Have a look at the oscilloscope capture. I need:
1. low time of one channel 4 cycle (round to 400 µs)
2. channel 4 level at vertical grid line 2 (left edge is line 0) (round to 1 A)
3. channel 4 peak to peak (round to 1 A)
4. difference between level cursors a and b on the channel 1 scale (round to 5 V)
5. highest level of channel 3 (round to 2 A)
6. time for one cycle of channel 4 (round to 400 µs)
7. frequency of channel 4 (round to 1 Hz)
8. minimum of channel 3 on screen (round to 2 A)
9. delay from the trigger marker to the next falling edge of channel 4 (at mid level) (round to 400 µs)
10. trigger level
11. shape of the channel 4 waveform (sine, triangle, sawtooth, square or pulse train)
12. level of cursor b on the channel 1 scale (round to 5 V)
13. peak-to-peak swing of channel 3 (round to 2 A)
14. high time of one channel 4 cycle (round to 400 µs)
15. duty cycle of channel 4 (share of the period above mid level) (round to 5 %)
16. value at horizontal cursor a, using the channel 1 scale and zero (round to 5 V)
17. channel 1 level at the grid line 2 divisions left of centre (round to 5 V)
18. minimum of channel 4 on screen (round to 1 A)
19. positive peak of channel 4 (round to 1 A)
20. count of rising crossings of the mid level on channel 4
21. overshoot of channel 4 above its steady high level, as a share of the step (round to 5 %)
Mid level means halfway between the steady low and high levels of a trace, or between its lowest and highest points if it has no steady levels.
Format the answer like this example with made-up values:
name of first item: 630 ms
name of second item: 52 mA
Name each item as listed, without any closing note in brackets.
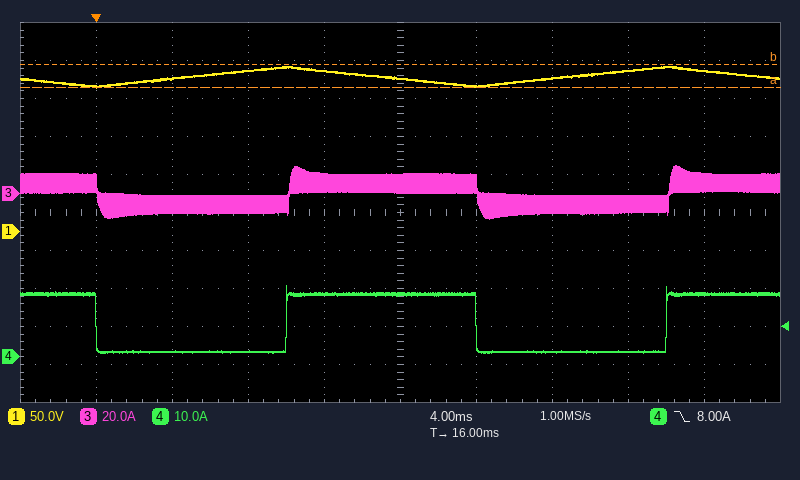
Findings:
low time of one channel 4 cycle: 10.0 ms
channel 4 level at vertical grid line 2 (left edge is line 0): 1 A
channel 4 peak to peak: 18 A
difference between level cursors a and b on the channel 1 scale: 30 V
highest level of channel 3: 14 A
time for one cycle of channel 4: 20.0 ms
frequency of channel 4: 50 Hz
minimum of channel 3 on screen: -14 A
delay from the trigger marker to the next falling edge of channel 4 (at mid level): 20.0 ms
trigger level: 8.00 A
shape of the channel 4 waveform: square
level of cursor b on the channel 1 scale: 220 V
peak-to-peak swing of channel 3: 28 A
high time of one channel 4 cycle: 10.0 ms
duty cycle of channel 4 (share of the period above mid level): 50 %
value at horizontal cursor a, using the channel 1 scale and zero: 190 V
channel 1 level at the grid line 2 divisions left of centre: 210 V
minimum of channel 4 on screen: 1 A
positive peak of channel 4: 19 A
count of rising crossings of the mid level on channel 4: 2
overshoot of channel 4 above its steady high level, as a share of the step: 15 %
